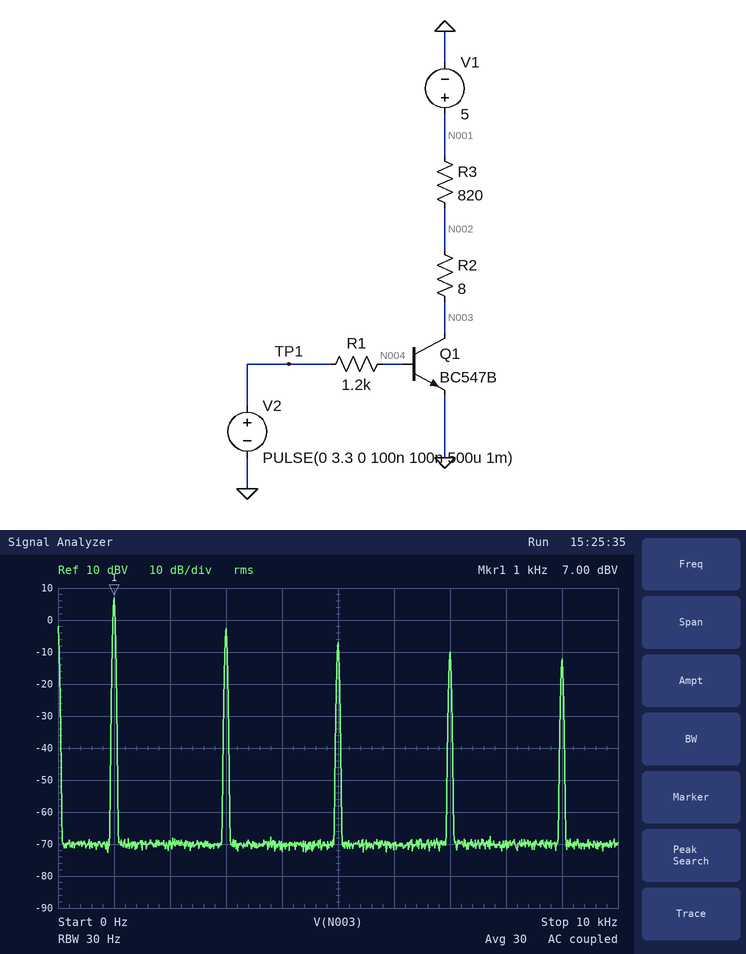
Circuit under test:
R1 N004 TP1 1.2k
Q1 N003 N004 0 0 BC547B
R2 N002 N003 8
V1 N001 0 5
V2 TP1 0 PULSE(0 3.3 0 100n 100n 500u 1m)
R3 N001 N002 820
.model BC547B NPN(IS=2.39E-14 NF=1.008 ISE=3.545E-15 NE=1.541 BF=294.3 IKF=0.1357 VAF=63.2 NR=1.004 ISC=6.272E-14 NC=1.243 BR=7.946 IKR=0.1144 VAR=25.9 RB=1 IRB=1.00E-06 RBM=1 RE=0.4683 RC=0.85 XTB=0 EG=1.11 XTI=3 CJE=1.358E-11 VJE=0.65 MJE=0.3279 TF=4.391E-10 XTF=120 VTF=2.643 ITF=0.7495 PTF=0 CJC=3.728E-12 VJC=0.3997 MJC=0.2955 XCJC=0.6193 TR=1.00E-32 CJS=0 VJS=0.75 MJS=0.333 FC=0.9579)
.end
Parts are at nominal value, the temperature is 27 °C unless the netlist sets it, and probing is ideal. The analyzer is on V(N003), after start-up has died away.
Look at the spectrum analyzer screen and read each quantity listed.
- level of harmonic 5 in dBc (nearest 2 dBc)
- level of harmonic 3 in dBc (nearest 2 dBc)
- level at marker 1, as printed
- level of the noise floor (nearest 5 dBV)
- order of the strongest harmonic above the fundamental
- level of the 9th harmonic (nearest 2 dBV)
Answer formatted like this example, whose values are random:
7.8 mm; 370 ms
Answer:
-14 dBc; -10 dBc; 7.00 dBV; -70 dBV; 3; -12 dBV
